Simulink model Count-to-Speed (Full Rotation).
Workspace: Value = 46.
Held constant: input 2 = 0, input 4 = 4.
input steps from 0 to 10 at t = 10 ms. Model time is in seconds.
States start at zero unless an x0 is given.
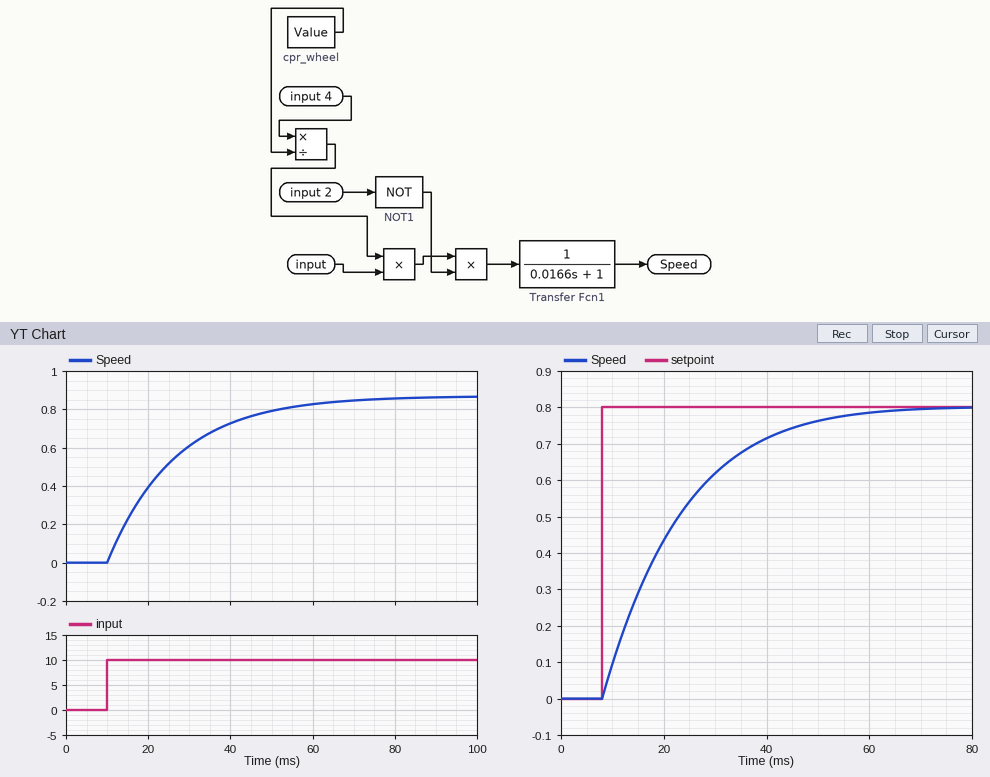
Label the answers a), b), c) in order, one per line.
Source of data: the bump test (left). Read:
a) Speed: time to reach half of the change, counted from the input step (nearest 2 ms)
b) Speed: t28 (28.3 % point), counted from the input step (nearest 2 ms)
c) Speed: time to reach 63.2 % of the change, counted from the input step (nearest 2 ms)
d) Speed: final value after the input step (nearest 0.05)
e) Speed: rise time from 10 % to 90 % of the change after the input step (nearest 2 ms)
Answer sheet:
a) 12 ms
b) 6 ms
c) 16 ms
d) 0.85
e) 36 ms
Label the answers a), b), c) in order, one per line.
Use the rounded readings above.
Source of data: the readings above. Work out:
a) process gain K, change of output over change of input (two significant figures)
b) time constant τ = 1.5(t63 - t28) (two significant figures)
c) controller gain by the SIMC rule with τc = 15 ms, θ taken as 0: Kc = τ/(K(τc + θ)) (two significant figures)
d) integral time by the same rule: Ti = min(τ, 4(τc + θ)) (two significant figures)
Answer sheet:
a) 0.085
b) 15 ms
c) 12
d) 15 ms
